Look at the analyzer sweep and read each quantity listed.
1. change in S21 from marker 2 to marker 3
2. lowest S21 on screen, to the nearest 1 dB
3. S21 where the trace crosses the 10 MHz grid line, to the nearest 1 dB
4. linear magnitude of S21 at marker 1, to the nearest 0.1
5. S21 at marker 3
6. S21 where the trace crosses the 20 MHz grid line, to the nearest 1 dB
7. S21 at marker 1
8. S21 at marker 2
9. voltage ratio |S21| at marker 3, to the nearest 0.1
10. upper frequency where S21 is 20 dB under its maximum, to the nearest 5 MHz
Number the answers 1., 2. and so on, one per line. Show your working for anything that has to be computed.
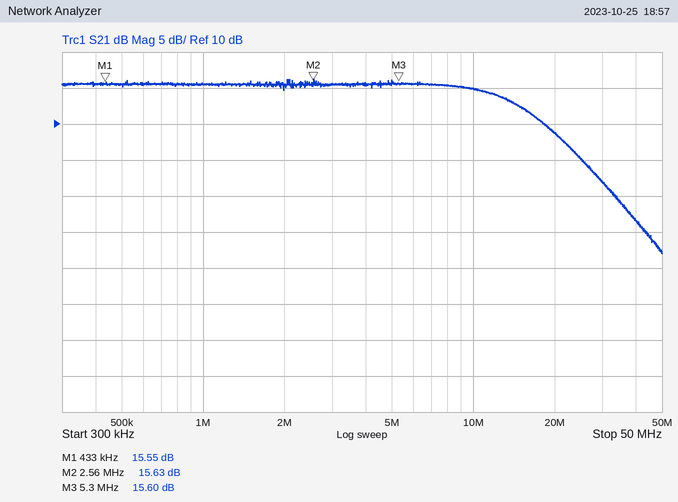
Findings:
1. 15.6 − (15.63) = -0.03 dB
2. -8 dB
3. 15 dB
4. 10^(15.55/20) ≈ 6.0
5. 15.60 dB
6. 9 dB
7. 15.55 dB
8. 15.63 dB
9. 10^(15.6/20) ≈ 6.0
10. 40 MHz
